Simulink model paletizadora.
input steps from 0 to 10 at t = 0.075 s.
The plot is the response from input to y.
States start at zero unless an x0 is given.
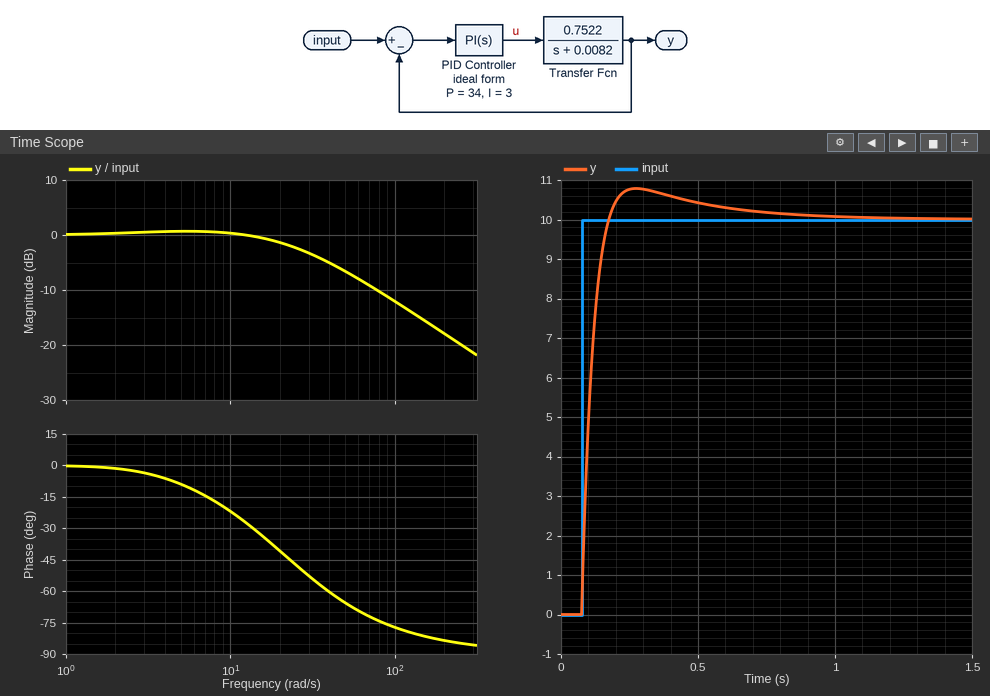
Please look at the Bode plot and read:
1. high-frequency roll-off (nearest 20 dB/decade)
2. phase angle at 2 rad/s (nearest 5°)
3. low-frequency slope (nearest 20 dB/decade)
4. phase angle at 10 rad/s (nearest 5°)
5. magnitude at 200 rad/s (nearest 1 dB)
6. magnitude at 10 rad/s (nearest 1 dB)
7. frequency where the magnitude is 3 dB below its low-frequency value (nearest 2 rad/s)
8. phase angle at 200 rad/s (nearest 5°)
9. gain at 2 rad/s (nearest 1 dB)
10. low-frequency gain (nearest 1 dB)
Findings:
-20 dB/decade
0°
0 dB/decade
-20°
-18 dB
0 dB
28 rad/s
-85°
0 dB
0 dB
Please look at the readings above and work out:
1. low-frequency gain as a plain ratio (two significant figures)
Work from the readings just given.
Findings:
1.0
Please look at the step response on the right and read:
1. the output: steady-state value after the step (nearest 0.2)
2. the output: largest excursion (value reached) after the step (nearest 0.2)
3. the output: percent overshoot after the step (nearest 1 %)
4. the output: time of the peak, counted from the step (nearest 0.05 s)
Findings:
10.0
10.8
8 %
0.20 s
